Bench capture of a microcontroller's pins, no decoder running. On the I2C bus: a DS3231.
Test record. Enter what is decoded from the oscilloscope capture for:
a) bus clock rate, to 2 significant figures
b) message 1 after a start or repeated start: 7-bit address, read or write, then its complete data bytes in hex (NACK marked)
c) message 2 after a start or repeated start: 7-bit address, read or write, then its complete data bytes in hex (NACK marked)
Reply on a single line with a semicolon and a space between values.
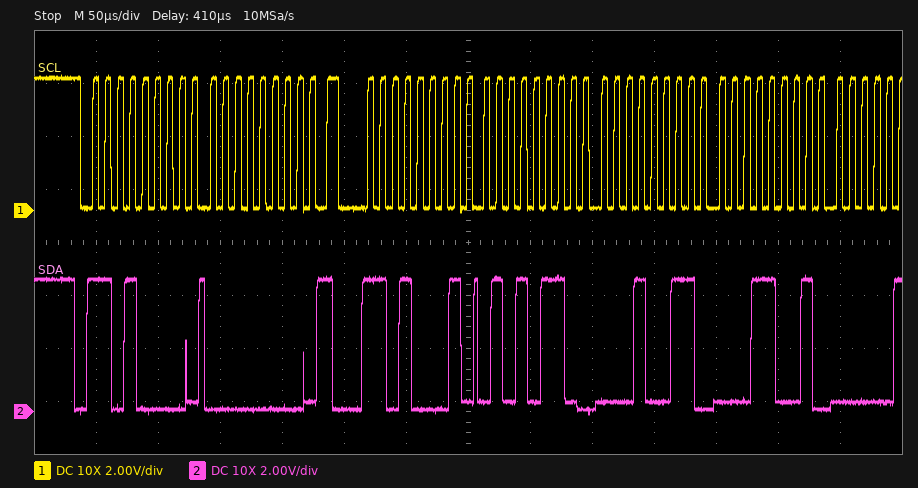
100 kHz; 0x68 write: 00; 0x68 read: 56 13 19
